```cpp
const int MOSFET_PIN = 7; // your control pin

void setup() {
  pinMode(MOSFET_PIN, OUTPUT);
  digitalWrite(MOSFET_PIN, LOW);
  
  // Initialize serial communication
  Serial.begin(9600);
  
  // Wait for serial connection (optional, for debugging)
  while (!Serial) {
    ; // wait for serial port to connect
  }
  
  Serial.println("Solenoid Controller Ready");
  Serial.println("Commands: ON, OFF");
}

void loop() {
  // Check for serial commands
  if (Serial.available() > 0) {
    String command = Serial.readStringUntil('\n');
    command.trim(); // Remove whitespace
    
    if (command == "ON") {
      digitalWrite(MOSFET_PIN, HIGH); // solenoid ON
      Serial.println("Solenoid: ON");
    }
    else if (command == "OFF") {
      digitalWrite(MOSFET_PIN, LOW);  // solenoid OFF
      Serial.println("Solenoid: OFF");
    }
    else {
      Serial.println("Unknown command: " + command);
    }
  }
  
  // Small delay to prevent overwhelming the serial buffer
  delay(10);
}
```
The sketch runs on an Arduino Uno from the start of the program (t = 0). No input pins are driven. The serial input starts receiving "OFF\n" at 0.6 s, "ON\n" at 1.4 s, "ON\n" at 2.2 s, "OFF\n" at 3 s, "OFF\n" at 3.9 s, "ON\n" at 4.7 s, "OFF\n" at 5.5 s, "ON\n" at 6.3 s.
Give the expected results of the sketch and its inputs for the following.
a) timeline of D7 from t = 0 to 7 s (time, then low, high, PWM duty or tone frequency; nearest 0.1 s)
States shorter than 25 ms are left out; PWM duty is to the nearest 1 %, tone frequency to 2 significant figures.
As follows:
0 s low; 1.4 s high; 3 s low; 4.7 s high; 5.5 s low; 6.3 s high
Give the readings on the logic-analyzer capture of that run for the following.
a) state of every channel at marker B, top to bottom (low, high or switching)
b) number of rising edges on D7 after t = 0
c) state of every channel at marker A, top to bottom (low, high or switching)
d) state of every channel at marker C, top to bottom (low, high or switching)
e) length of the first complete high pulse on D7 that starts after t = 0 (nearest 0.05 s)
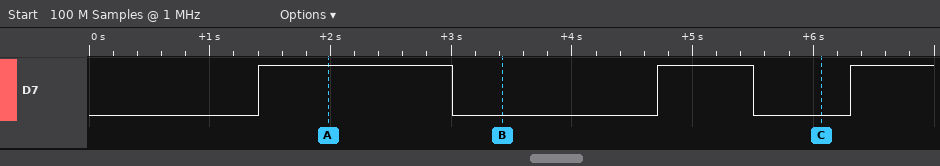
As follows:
D7 low
3
D7 high
D7 low
1.60 s
